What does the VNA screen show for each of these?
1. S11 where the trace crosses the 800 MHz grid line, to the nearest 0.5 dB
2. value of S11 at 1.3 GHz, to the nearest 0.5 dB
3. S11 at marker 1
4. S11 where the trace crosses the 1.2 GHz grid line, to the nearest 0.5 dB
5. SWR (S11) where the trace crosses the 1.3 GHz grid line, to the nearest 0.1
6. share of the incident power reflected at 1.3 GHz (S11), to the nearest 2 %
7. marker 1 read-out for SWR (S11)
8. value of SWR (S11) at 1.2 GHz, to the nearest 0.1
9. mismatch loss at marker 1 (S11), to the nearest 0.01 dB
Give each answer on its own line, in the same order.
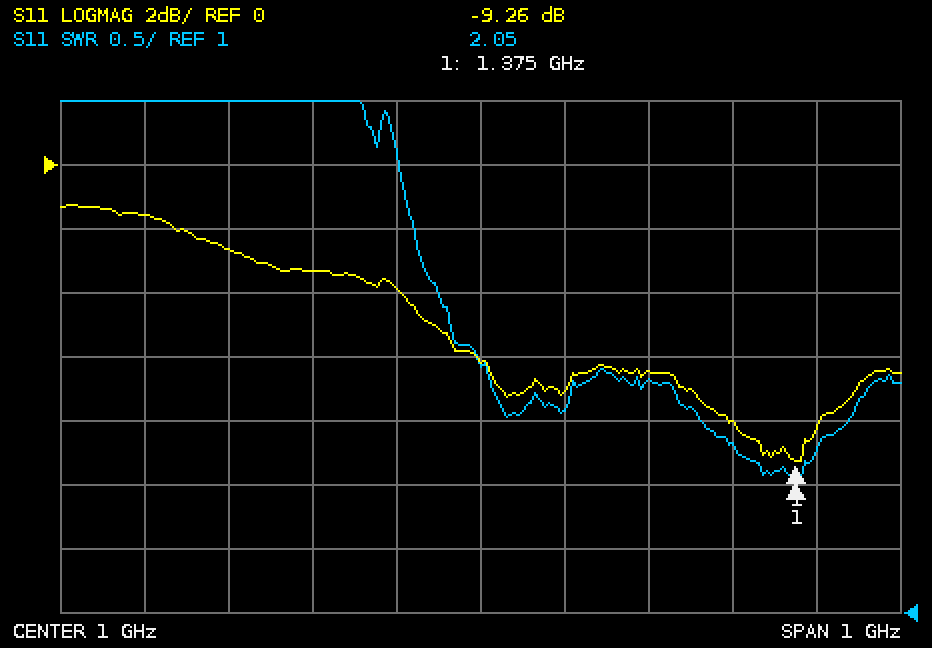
-3.5 dB
-8.0 dB
-9.26 dB
-6.5 dB
2.3
16 %
2.05
2.8
0.55 dB
